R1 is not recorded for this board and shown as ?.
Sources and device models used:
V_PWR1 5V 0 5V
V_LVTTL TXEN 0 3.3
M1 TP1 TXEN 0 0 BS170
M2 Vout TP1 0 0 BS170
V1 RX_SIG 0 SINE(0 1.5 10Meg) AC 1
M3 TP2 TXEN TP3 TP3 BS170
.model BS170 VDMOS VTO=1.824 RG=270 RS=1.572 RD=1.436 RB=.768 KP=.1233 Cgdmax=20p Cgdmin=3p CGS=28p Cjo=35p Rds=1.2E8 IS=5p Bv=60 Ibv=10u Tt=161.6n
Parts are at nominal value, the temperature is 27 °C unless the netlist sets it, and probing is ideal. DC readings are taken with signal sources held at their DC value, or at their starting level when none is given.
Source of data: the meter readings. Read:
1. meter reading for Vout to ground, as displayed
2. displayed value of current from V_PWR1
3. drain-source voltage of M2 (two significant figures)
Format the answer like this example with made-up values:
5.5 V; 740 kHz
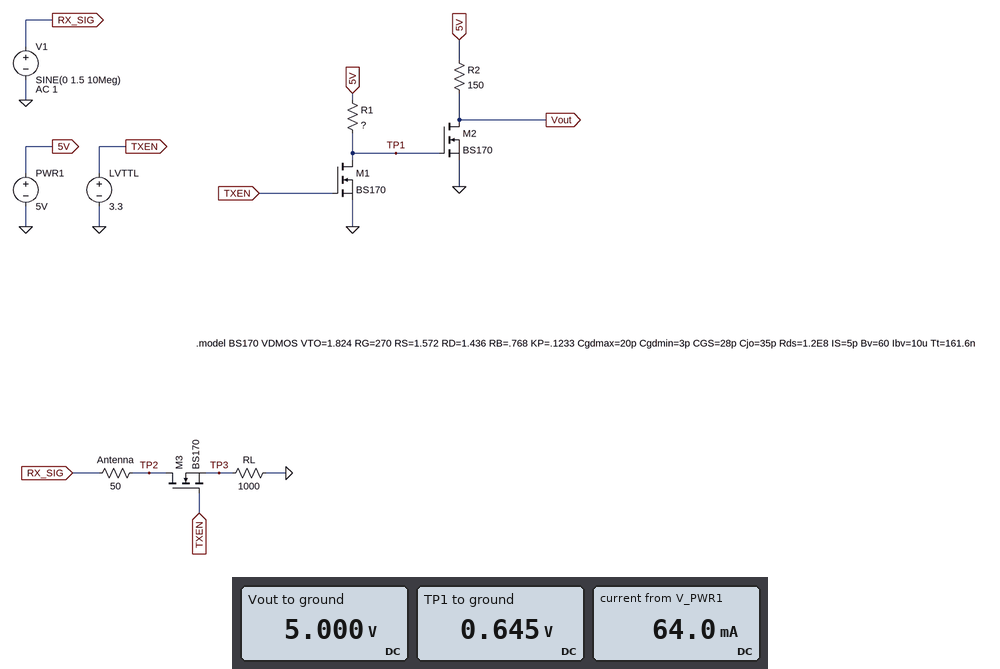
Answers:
5.000 V; 64.0 mA; 5.0 V
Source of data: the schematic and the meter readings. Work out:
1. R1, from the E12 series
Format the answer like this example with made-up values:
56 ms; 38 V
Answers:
68 Ω
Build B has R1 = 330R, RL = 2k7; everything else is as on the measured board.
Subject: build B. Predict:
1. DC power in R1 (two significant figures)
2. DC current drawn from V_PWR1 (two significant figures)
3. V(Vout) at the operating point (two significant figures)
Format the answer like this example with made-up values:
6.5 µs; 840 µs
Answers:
72 mW; 15 mA; 5.0 V
